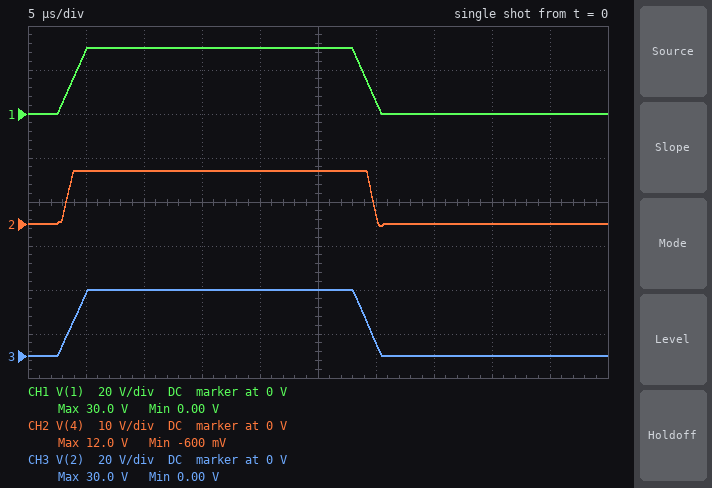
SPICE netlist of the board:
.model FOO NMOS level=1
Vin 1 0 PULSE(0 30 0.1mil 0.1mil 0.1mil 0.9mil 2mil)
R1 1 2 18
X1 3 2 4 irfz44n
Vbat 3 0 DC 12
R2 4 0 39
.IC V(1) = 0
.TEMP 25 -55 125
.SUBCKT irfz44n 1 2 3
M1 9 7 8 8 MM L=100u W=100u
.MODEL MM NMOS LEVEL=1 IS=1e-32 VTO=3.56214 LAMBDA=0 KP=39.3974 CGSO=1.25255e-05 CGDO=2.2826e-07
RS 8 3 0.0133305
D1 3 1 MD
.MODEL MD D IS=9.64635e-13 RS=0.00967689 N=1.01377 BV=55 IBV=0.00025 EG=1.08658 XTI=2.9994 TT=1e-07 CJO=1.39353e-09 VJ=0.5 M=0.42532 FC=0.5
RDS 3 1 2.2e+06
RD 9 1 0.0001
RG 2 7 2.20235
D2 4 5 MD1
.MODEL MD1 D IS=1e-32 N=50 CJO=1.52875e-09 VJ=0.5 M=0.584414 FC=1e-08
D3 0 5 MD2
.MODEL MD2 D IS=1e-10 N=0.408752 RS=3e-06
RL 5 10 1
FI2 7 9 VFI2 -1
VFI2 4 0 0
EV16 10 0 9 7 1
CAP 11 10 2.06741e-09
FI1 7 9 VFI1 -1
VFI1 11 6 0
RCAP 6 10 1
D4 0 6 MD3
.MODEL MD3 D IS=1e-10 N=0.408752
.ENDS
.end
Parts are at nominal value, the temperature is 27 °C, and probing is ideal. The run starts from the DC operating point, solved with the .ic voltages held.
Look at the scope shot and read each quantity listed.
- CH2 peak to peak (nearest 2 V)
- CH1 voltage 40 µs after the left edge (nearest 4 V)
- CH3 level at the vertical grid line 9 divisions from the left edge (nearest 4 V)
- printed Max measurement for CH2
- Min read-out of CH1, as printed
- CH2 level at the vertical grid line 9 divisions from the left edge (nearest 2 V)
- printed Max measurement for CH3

12 V
0 V
0 V
12.0 V
0.00 V
0 V
30.0 V
